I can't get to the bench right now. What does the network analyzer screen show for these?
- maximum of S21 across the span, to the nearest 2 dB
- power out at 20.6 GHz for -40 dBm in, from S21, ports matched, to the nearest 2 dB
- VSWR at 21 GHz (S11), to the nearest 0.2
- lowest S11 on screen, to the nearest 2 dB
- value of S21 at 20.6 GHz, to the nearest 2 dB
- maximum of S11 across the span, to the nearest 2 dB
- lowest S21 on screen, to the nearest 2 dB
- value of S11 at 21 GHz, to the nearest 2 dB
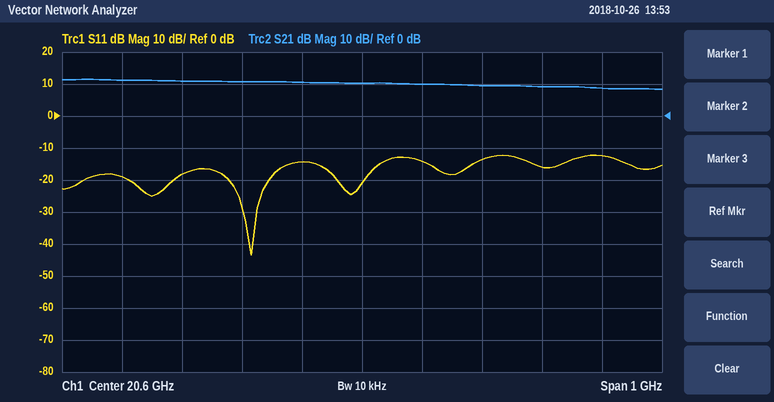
12 dB
-30 dBm
1.6
-44 dB
10 dB
-12 dB
8 dB
-12 dB
